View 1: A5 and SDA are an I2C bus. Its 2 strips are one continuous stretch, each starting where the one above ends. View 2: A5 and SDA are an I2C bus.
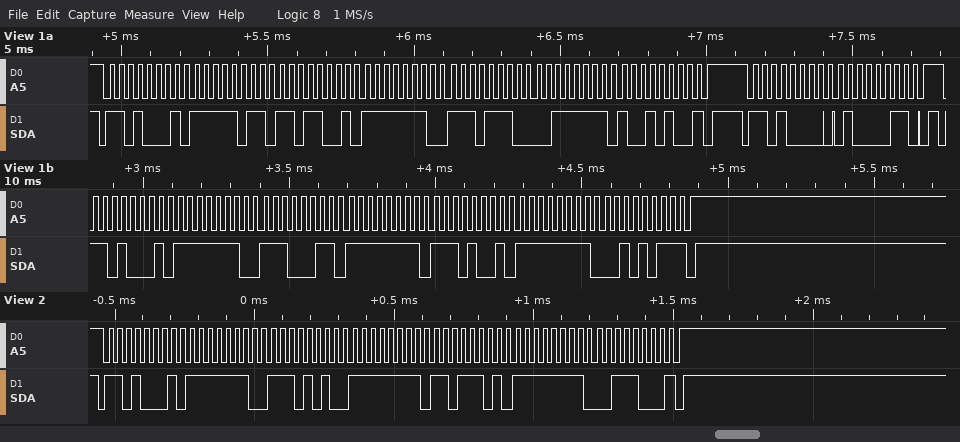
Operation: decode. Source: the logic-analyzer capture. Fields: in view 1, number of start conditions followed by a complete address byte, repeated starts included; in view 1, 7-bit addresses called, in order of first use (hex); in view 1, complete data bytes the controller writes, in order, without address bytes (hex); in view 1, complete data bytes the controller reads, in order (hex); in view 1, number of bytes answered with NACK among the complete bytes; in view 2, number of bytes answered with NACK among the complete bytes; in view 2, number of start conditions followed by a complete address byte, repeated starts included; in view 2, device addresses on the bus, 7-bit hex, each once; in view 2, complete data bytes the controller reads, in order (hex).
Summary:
3
0x68
43
FB D9 FE EE 3F 94 FE E3 FF E9 FF 2B
2
1
1
0x68
FE EA FF DD FF 38
